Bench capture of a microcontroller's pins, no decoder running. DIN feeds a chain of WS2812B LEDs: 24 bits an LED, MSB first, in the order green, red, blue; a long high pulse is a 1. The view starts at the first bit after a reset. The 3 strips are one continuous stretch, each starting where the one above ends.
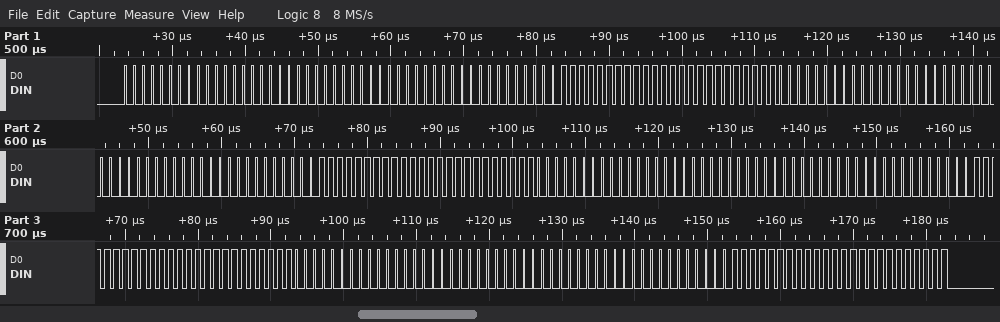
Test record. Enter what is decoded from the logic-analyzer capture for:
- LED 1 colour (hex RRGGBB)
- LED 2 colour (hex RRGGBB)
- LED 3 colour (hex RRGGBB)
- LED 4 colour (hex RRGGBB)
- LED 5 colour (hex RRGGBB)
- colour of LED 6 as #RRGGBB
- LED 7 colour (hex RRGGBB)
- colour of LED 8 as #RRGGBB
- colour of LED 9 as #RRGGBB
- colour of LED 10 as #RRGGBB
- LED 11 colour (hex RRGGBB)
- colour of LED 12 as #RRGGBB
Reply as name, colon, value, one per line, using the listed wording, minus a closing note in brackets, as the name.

LED 1 colour: #000000
LED 2 colour: #000000
LED 3 colour: #FFFFFF
LED 4 colour: #000000
LED 5 colour: #000000
colour of LED 6 as #RRGGBB: #FFFFFF
LED 7 colour: #000000
colour of LED 8 as #RRGGBB: #000000
colour of LED 9 as #RRGGBB: #FFFFFF
colour of LED 10 as #RRGGBB: #000000
LED 11 colour: #000000
colour of LED 12 as #RRGGBB: #FFFFFF
